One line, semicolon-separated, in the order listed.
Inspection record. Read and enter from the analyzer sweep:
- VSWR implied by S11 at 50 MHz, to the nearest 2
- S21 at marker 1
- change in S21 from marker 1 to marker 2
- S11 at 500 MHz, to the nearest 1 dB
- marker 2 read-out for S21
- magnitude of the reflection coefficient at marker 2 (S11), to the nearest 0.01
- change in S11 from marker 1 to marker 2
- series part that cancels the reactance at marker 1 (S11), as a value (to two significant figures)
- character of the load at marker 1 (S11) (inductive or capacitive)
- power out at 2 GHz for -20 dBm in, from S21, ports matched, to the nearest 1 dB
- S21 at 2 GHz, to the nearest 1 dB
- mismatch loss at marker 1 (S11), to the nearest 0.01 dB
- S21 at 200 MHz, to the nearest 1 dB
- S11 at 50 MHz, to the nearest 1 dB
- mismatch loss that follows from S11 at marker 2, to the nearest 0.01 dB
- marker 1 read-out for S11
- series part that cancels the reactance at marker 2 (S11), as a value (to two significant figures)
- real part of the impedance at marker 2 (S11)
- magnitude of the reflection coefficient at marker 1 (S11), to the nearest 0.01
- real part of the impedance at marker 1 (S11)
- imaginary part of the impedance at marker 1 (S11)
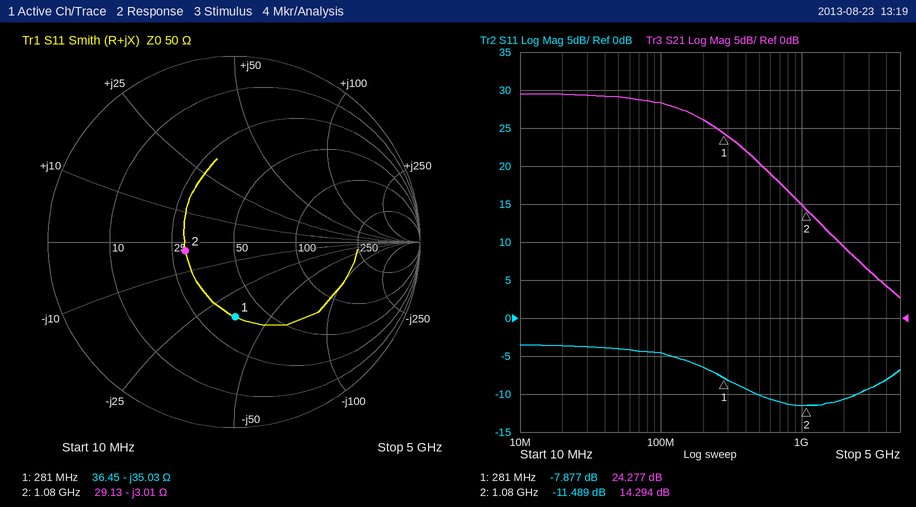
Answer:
4; 24.277 dB; -9.983 dB; -10 dB; 14.294 dB; 0.27; -3.612 dB; 20 nH; capacitive; -11 dBm; 9 dB; 0.77 dB; 26 dB; -4 dB; 0.32 dB; -7.877 dB; 440 pH; 29.13 Ω; 0.40; 36.45 Ω; -35.03 Ω
